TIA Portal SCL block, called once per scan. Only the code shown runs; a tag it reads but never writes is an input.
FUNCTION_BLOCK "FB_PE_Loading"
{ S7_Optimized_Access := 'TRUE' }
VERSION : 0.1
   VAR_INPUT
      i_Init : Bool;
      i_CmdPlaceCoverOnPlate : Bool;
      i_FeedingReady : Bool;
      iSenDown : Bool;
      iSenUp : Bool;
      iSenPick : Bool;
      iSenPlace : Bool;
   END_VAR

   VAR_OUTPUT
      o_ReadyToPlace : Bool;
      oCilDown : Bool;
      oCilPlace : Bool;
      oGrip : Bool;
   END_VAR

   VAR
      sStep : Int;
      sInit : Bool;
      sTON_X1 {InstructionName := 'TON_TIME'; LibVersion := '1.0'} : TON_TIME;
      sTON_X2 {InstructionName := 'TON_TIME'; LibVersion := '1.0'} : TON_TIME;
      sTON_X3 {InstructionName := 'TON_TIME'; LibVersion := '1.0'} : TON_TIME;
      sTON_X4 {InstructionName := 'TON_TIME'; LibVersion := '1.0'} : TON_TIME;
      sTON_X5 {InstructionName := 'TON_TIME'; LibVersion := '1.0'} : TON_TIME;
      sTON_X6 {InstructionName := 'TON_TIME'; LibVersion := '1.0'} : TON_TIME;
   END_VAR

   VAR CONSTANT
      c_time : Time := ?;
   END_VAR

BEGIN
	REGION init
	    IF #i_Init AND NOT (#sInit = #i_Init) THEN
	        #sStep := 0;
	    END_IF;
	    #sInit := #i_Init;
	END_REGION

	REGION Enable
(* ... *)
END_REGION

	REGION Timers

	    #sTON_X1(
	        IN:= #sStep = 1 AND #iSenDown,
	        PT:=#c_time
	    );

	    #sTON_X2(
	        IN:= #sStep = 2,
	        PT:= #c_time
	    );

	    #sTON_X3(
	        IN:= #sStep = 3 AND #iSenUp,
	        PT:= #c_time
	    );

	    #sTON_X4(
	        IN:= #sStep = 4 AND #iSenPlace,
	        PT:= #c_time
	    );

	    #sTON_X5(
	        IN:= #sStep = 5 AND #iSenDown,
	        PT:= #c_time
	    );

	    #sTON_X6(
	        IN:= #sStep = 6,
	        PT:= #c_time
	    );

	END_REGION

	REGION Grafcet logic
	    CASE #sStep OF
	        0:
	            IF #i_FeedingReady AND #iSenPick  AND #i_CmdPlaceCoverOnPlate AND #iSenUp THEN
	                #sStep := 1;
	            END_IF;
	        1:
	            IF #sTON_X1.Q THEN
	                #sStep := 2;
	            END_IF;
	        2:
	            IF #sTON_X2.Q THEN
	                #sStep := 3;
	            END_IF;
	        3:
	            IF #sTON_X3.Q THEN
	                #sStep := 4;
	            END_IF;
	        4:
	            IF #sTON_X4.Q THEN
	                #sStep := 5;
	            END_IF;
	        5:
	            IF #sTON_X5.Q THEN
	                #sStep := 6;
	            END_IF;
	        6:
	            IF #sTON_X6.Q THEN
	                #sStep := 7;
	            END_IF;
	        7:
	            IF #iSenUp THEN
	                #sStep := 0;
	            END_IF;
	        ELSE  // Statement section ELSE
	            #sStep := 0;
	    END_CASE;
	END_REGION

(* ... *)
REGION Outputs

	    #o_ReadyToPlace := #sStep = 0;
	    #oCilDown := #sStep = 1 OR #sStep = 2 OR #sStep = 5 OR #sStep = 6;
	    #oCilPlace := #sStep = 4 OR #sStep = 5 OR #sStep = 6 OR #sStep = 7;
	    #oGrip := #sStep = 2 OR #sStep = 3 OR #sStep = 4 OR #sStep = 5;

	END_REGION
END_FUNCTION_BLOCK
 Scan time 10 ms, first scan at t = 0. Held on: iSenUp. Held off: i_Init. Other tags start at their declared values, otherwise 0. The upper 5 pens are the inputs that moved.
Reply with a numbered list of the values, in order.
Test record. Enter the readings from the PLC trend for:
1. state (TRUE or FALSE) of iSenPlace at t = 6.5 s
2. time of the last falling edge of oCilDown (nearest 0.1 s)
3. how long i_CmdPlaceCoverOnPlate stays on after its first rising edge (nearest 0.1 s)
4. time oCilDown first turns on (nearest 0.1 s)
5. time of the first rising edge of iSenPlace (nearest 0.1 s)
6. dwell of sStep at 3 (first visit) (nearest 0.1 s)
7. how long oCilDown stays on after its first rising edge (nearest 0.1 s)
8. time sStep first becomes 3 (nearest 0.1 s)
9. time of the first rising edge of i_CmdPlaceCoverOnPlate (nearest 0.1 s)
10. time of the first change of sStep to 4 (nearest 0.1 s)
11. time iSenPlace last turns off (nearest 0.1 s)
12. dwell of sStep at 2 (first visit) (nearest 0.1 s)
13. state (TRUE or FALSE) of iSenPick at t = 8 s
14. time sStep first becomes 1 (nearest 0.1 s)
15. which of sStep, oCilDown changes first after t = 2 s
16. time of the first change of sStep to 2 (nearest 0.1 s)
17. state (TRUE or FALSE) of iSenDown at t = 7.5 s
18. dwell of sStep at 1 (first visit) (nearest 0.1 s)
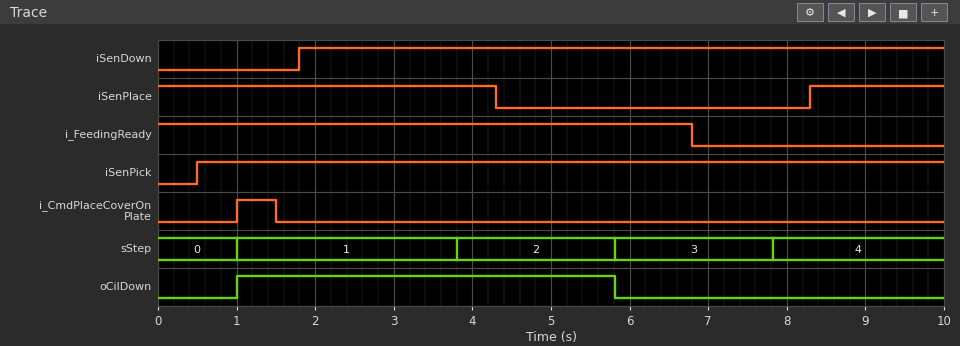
1. FALSE
2. 5.8 s
3. 0.5 s
4. 1.0 s
5. 8.3 s
6. 2.0 s
7. 4.8 s
8. 5.8 s
9. 1.0 s
10. 7.8 s
11. 4.3 s
12. 2.0 s
13. TRUE
14. 1.0 s
15. sStep
16. 3.8 s
17. TRUE
18. 2.8 s
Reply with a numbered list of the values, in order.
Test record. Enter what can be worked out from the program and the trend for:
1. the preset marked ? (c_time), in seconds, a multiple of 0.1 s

1. 2.0 s
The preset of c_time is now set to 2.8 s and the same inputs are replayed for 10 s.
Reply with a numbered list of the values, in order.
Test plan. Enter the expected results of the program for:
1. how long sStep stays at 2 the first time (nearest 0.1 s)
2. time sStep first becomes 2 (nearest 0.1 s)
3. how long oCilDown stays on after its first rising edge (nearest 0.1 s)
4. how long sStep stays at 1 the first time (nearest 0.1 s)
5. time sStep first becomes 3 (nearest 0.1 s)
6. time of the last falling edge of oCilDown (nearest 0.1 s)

1. 2.8 s
2. 4.6 s
3. 6.4 s
4. 3.6 s
5. 7.4 s
6. 7.4 s
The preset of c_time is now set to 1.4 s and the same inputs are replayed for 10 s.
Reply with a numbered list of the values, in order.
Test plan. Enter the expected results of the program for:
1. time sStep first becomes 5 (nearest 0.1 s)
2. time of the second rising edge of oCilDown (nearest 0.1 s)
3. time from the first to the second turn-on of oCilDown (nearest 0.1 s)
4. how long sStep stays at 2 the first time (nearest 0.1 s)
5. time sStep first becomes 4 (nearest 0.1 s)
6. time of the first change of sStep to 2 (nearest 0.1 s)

1. 9.7 s
2. 9.7 s
3. 8.7 s
4. 1.4 s
5. 6.0 s
6. 3.2 s
